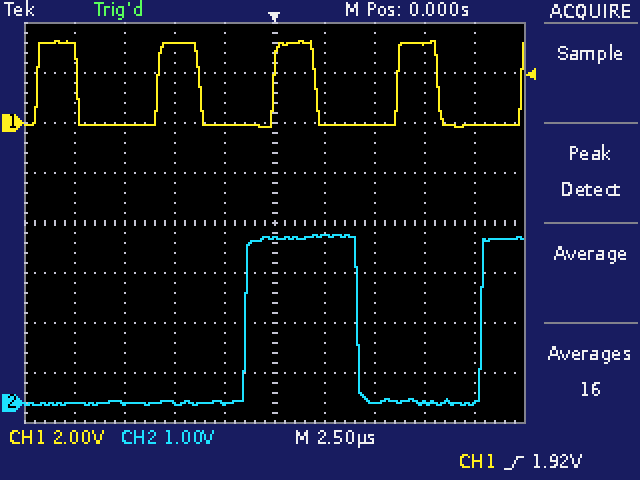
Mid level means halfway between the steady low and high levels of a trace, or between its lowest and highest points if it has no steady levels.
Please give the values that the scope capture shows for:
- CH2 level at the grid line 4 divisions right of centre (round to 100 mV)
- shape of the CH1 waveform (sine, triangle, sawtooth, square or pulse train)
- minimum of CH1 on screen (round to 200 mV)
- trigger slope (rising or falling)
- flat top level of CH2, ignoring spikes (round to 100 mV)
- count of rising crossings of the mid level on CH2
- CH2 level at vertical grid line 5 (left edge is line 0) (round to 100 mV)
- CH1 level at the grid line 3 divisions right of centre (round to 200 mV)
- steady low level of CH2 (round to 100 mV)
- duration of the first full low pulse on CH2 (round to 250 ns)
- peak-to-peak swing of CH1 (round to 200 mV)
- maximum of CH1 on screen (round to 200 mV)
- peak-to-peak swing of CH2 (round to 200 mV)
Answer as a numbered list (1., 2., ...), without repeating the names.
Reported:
1. 0.0 V
2. pulse train
3. -200 mV
4. rising
5. 3.3 V
6. 2
7. 3.3 V
8. 3.2 V
9. 0.0 V
10. 6.25 µs
11. 3.4 V
12. 3.2 V
13. 3.4 V
